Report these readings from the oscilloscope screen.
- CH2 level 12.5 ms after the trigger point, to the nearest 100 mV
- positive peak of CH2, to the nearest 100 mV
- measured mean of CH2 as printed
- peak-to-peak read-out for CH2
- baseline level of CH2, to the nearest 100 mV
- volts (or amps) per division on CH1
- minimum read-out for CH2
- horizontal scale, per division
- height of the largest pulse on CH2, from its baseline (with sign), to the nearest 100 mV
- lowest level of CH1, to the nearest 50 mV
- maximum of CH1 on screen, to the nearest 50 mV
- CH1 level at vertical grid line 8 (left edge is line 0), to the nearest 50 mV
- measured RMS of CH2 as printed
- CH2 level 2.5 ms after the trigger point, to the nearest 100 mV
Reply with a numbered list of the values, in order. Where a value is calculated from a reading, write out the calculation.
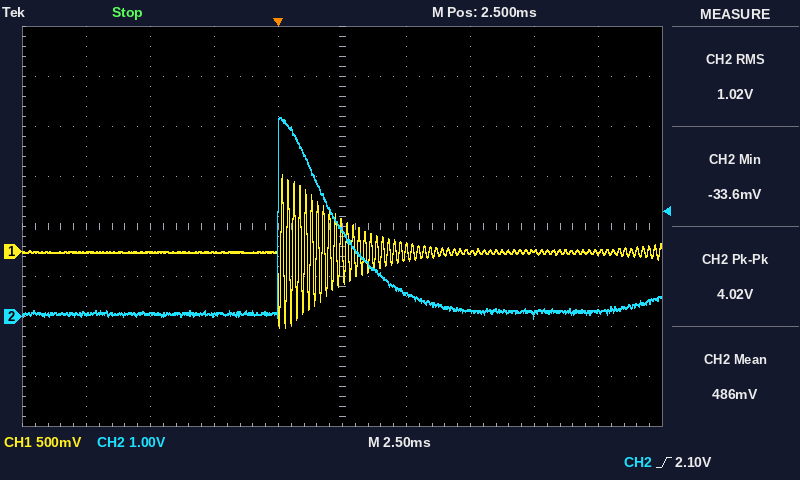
1. 100 mV
2. 4.0 V
3. 486 mV
4. 4.02 V
5. 100 mV
6. 500 mV
7. -33.6 mV
8. 2.5 ms
9. 4.0 V − (100 mV) = +3.9 V
10. -750 mV
11. 750 mV
12. 0 mV
13. 1.02 V
14. 1.7 V
